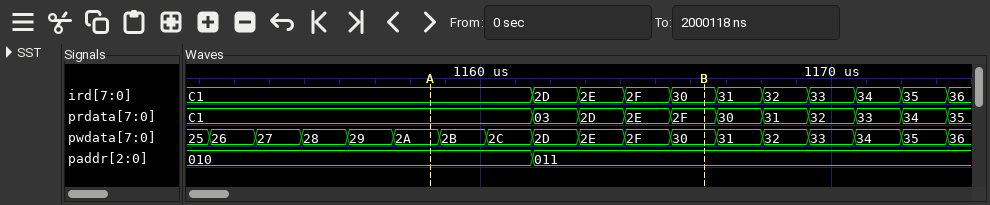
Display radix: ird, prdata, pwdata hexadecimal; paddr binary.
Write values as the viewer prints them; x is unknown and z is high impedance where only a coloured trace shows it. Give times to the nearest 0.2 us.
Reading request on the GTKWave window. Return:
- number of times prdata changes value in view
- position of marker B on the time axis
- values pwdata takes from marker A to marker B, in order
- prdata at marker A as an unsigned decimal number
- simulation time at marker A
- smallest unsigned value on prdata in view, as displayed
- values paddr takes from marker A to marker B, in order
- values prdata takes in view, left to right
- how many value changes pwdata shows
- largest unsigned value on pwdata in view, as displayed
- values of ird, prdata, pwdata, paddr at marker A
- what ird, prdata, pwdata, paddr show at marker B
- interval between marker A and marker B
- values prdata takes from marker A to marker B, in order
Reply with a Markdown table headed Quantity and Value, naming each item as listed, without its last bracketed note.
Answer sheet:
| Quantity | Value |
|---|---|
| number of times prdata changes value in view | 10 |
| position of marker B on the time axis | 1166.4 us |
| values pwdata takes from marker A to marker B, in order | 2A, 2B, 2C, 2D, 2E, 2F, 30 |
| prdata at marker A as an unsigned decimal number | 193 |
| simulation time at marker A | 1158.6 us |
| smallest unsigned value on prdata in view, as displayed | 03 |
| values paddr takes from marker A to marker B, in order | 010, 011 |
| values prdata takes in view, left to right | C1, 03, 2D, 2E, 2F, 30, 31, 32, 33, 34, 35 |
| how many value changes pwdata shows | 17 |
| largest unsigned value on pwdata in view, as displayed | 36 |
| values of ird, prdata, pwdata, paddr at marker A | ird=C1, prdata=C1, pwdata=2A, paddr=010 |
| what ird, prdata, pwdata, paddr show at marker B | ird=30, prdata=2F, pwdata=30, paddr=011 |
| interval between marker A and marker B | 7.8 us |
| values prdata takes from marker A to marker B, in order | C1, 03, 2D, 2E, 2F |
